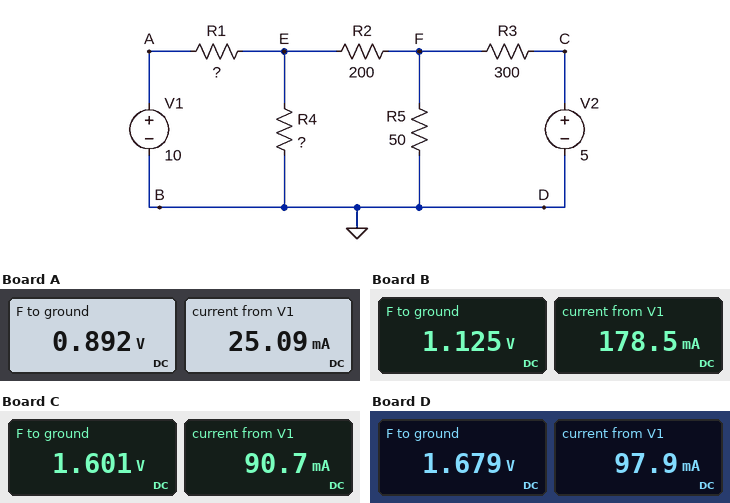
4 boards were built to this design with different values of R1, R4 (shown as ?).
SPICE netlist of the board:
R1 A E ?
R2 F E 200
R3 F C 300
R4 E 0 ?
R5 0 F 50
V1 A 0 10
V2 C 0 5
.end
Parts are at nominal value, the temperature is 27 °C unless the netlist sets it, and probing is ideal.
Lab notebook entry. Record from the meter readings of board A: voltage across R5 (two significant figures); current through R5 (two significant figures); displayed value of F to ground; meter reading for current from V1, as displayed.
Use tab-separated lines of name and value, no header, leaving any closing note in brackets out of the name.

voltage across R5	890 mV
current through R5	18 mA
displayed value of F to ground	0.892 V
meter reading for current from V1, as displayed	25.09 mA
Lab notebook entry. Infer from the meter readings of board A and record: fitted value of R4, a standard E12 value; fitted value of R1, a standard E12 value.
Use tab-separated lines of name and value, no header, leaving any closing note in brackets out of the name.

fitted value of R4, a standard E12 value	82 Ω
fitted value of R1, a standard E12 value	330 Ω
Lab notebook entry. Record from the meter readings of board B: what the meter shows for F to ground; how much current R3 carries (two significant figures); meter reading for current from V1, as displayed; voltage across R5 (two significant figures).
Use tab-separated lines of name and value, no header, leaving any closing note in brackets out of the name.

what the meter shows for F to ground	1.125 V
how much current R3 carries	13 mA
meter reading for current from V1, as displayed	178.5 mA
voltage across R5	1.1 V
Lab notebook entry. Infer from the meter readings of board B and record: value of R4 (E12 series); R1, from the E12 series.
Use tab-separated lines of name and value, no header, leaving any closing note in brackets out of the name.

value of R4	18 Ω
R1, from the E12 series	39 Ω
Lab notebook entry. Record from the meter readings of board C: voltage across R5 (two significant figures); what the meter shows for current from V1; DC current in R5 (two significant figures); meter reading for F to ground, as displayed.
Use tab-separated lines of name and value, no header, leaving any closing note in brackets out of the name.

voltage across R5	1.6 V
what the meter shows for current from V1	90.7 mA
DC current in R5	32 mA
meter reading for F to ground, as displayed	1.601 V
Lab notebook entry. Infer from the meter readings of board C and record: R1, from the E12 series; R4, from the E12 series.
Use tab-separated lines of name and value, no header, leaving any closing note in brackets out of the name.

R1, from the E12 series	47 Ω
R4, from the E12 series	82 Ω
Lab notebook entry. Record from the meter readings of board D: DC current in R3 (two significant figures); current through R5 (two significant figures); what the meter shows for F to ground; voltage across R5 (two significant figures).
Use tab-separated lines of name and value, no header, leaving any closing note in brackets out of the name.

DC current in R3	11 mA
current through R5	34 mA
what the meter shows for F to ground	1.679 V
voltage across R5	1.7 V
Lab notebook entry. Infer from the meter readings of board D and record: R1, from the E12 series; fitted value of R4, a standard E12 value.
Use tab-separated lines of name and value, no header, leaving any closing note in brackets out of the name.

R1, from the E12 series	39 Ω
fitted value of R4, a standard E12 value	82 Ω
